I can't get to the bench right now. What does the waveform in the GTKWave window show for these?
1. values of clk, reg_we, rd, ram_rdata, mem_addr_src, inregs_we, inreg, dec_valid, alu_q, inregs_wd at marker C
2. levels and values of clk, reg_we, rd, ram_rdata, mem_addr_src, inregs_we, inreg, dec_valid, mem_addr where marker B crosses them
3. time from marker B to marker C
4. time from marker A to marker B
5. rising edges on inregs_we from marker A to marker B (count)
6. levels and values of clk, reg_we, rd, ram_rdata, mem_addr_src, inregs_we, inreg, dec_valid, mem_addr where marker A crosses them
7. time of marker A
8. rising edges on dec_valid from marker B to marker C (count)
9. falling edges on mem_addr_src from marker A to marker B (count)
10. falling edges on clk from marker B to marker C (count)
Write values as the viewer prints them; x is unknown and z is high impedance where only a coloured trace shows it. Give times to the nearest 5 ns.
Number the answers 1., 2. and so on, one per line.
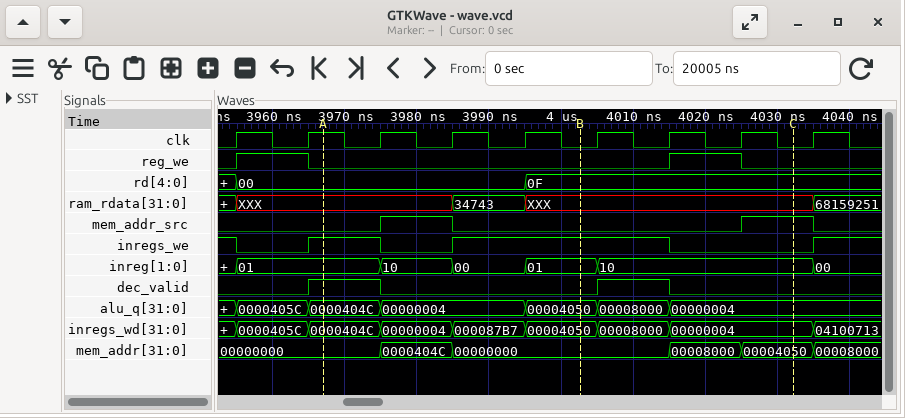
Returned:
1. clk=0, reg_we=0, rd=0F, ram_rdata=XXX, mem_addr_src=1, inregs_we=0, inreg=10, dec_valid=0, alu_q=00000004, inregs_wd=00000004
2. clk=0, reg_we=0, rd=0F, ram_rdata=XXX, mem_addr_src=0, inregs_we=1, inreg=01, dec_valid=0, mem_addr=00000000
3. 30 ns
4. 35 ns
5. 1
6. clk=1, reg_we=0, rd=00, ram_rdata=XXX, mem_addr_src=0, inregs_we=1, inreg=01, dec_valid=1, mem_addr=00000000
7. 3965 ns
8. 1
9. 1
10. 3
